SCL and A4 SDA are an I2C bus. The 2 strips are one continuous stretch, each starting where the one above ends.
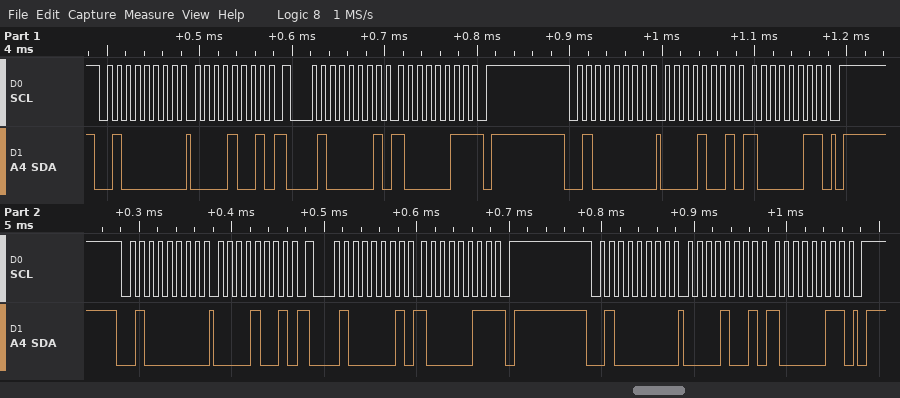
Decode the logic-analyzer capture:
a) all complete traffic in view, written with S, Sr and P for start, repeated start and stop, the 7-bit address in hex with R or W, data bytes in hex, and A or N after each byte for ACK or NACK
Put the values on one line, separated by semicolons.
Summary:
S 20W A 09 A Sr 20R A 83 N P S 20W A 09 A 83 A P S 20W A 09 A Sr 20R A 83 N P S 20W A 09 A 83 A P
